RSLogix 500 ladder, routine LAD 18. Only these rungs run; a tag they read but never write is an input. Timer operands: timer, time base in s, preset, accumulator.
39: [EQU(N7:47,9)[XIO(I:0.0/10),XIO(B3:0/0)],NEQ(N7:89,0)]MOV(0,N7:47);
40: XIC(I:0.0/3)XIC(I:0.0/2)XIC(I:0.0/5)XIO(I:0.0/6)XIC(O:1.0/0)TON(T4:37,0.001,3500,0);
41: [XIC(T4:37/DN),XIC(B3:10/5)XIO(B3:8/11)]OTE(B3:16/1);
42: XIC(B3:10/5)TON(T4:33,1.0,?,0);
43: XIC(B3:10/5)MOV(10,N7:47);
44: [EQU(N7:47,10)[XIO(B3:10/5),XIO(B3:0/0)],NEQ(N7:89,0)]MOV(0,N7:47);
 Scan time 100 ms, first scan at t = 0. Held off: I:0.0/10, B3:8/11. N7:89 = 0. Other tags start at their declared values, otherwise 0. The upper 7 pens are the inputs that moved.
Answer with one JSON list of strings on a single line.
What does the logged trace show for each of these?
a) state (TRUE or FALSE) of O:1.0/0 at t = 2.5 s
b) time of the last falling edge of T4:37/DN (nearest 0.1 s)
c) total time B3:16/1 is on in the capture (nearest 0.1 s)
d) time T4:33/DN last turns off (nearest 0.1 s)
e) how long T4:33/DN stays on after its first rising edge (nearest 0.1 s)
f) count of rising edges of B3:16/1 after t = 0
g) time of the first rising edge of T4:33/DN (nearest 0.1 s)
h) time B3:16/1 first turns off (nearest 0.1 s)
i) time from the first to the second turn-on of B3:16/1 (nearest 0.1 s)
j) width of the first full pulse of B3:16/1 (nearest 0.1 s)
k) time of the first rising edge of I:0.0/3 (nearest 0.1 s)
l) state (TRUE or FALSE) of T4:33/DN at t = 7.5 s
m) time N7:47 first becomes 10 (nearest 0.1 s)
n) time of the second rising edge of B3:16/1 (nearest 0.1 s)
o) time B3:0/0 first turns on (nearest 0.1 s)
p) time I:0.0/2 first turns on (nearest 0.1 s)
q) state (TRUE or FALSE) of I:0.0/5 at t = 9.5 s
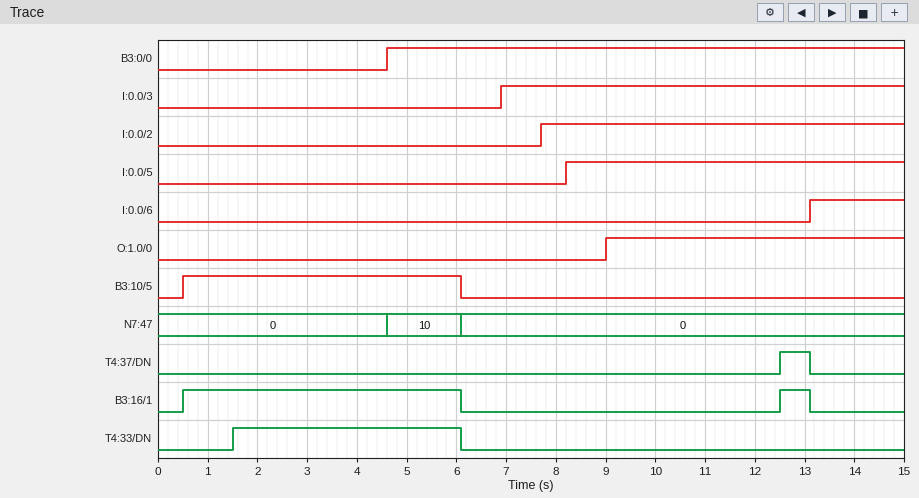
["FALSE", "13.1 s", "6.2 s", "6.1 s", "4.6 s", "2", "1.5 s", "6.1 s", "12.0 s", "5.6 s", "6.9 s", "FALSE", "4.6 s", "12.5 s", "4.6 s", "7.7 s", "TRUE"]
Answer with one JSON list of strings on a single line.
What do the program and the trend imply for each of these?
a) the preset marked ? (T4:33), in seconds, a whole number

["1 s"]
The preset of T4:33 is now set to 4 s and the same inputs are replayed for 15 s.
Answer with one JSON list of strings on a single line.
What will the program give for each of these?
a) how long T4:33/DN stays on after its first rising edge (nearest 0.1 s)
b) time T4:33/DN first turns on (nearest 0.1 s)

["1.6 s", "4.5 s"]
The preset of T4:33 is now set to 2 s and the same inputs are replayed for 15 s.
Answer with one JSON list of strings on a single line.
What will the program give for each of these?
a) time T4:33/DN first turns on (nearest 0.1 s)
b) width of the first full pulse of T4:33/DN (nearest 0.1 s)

["2.5 s", "3.6 s"]
